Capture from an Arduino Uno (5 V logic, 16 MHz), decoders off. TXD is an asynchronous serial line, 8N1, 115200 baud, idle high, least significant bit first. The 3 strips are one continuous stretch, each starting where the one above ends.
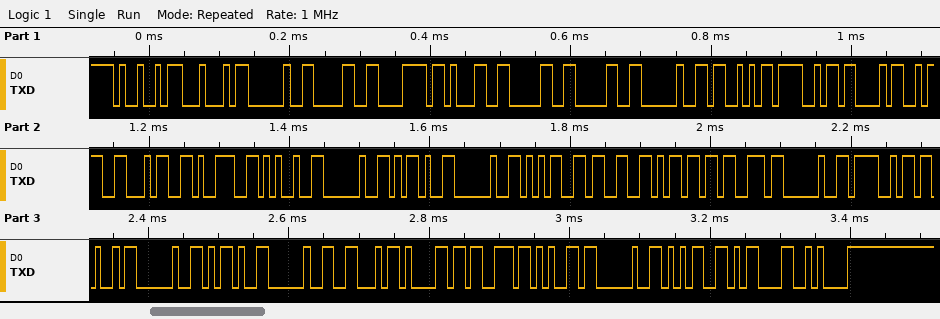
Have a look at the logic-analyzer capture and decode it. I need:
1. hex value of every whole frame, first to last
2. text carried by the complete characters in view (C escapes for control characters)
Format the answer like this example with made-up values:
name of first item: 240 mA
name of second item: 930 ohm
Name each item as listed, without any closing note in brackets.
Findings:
hex value of every whole frame, first to last: 0x49 0x44 0x20 0x30 0x78 0x31 0x30 0x30 0x20 0x53 0x4F 0x43 0x3A 0x34 0x39 0x25 0x20 0x2D 0x20 0x35 0x33 0x6D 0x73 0x20 0x4F 0x4B 0x20 0x2D 0x20 0x46 0x61 0x73 0x65 0x20 0x35 0x0D 0x0A
text carried by the complete characters in view: "ID 0x100 SOC:49% - 53ms OK - Fase 5\r\n"
